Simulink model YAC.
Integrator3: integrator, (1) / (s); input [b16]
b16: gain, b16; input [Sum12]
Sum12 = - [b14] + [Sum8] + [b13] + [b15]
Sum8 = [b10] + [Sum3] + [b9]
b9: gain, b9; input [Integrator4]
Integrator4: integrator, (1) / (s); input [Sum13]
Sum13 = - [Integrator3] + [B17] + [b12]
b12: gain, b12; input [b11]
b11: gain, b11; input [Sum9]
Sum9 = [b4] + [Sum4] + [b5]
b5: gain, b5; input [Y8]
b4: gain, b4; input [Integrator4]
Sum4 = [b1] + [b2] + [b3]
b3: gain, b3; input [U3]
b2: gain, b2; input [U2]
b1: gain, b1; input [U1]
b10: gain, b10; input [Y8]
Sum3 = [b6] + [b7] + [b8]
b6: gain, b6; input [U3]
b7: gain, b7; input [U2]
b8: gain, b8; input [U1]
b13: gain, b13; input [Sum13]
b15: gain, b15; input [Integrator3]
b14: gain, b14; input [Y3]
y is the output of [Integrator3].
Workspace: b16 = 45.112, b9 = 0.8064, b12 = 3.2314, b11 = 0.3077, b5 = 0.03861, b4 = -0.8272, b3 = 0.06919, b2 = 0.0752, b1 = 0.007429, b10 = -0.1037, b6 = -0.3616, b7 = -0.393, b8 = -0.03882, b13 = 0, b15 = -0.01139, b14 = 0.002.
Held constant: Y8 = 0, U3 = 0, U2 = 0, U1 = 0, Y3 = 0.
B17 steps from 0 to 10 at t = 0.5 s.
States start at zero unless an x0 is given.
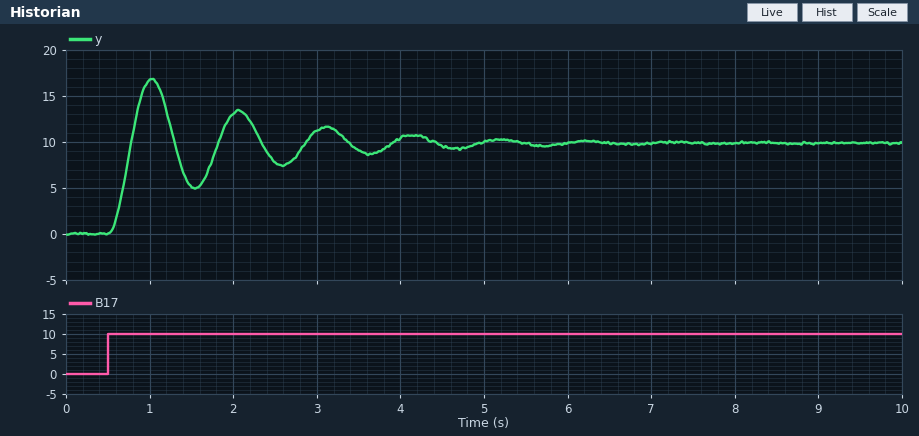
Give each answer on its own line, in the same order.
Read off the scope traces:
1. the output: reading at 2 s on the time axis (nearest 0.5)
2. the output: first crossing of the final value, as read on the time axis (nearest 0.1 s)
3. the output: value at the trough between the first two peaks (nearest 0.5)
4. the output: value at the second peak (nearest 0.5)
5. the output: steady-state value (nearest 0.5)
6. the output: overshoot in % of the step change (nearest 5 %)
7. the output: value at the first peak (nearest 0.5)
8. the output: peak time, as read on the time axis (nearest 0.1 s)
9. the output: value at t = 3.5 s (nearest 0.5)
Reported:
13.0
0.8 s
5.0
13.5
10.0
70 %
17.0
1.0 s
9.0
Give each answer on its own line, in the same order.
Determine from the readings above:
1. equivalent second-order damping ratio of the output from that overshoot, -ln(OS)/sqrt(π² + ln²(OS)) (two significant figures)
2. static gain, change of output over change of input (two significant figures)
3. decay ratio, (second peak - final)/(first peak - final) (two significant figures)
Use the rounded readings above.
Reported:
0.11
1.0
0.50
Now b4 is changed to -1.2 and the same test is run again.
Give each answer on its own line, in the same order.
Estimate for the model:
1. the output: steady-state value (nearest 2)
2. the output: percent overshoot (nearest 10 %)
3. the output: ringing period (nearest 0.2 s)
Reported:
10
60 %
1.0 s
